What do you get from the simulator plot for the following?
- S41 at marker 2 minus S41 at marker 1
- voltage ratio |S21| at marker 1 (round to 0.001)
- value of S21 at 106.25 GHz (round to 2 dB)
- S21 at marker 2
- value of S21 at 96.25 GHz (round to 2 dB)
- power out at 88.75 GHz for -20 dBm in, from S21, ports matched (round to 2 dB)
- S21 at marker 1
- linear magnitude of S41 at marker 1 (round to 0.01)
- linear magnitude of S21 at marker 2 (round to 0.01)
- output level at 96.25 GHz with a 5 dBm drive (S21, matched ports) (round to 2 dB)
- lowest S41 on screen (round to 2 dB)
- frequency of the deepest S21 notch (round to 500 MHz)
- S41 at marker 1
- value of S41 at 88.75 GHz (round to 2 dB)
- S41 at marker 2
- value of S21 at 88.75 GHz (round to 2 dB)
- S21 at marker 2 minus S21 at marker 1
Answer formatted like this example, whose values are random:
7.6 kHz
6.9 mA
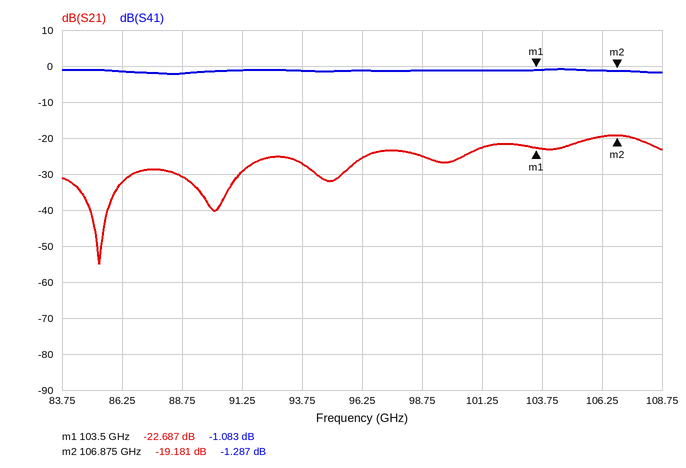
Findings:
-0.204 dB
0.073
-20 dB
-19.181 dB
-26 dB
-50 dBm
-22.687 dB
0.88
0.11
-20 dBm
-2 dB
85.5 GHz
-1.083 dB
-2 dB
-1.287 dB
-30 dB
3.506 dB
